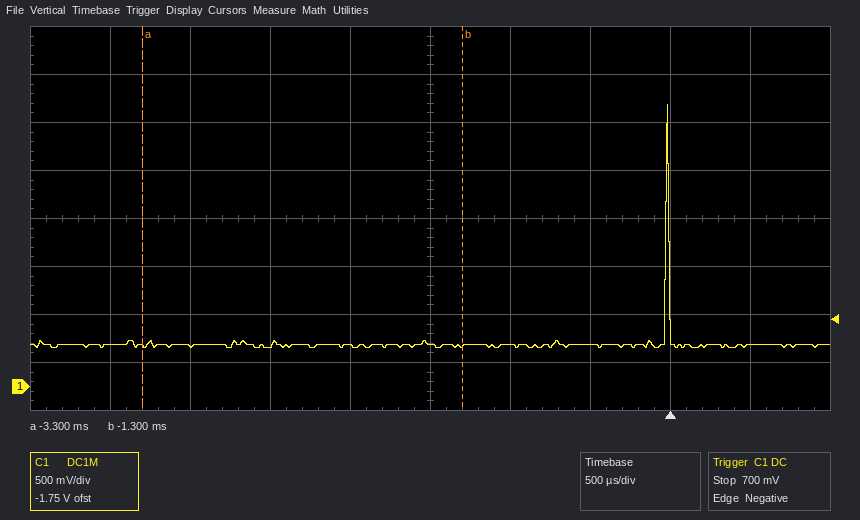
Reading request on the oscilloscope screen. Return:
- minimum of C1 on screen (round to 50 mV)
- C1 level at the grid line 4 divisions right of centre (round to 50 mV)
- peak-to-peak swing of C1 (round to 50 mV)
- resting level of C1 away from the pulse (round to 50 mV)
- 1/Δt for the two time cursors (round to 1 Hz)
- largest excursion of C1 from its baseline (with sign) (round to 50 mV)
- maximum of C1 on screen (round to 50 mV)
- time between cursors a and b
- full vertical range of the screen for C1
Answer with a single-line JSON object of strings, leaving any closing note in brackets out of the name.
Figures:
{"minimum of C1 on screen": "400 mV", "C1 level at the grid line 4 divisions right of centre": "450 mV", "peak-to-peak swing of C1": "2.55 V", "resting level of C1 away from the pulse": "450 mV", "1/Δt for the two time cursors": "500 Hz", "largest excursion of C1 from its baseline (with sign)": "+2.50 V", "maximum of C1 on screen": "2.95 V", "time between cursors a and b": "2.00 ms", "full vertical range of the screen for C1": "4 V"}
